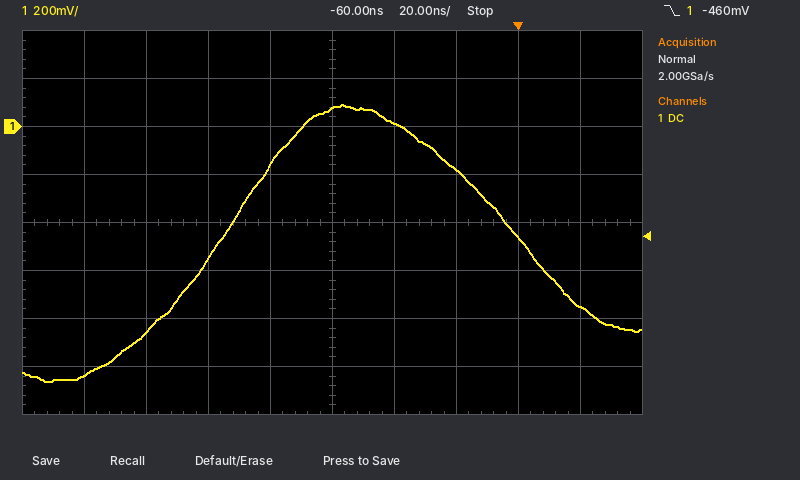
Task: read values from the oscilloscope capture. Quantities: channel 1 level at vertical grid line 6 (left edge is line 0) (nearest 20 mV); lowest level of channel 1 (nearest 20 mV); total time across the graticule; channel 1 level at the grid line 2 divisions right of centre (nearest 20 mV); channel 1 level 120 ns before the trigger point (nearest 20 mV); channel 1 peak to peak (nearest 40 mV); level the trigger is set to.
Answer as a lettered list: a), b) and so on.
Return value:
a) 20 mV
b) -1.06 V
c) 200 ns
d) -180 mV
e) -860 mV
f) 1.16 V
g) -460 mV
